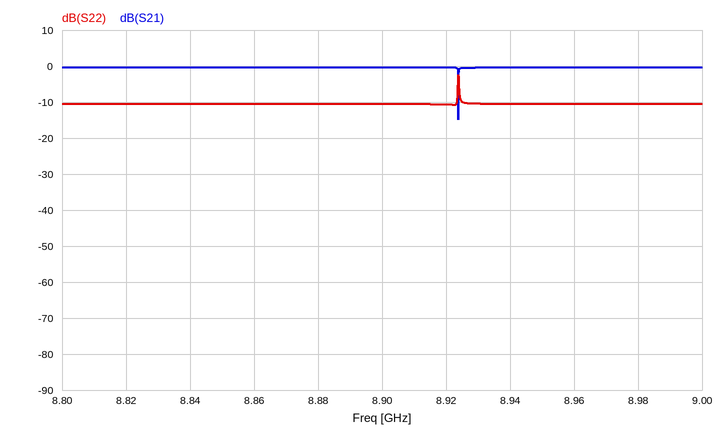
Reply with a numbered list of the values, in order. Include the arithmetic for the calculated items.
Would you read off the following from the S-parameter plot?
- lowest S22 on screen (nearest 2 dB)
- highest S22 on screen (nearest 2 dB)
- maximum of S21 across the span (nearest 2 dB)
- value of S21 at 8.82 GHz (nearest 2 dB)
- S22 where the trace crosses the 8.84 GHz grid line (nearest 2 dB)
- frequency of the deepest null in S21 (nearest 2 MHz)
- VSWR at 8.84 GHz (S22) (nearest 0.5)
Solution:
1. -10 dB
2. -2 dB
3. 0 dB
4. 0 dB
5. -10 dB
6. 8.924 GHz
7. |Γ| = 10^(-10/20) = 0.3162; VSWR = (1 + 0.3162)/(1 − 0.3162) ≈ 1.92, so 2.0 to the nearest 0.5
